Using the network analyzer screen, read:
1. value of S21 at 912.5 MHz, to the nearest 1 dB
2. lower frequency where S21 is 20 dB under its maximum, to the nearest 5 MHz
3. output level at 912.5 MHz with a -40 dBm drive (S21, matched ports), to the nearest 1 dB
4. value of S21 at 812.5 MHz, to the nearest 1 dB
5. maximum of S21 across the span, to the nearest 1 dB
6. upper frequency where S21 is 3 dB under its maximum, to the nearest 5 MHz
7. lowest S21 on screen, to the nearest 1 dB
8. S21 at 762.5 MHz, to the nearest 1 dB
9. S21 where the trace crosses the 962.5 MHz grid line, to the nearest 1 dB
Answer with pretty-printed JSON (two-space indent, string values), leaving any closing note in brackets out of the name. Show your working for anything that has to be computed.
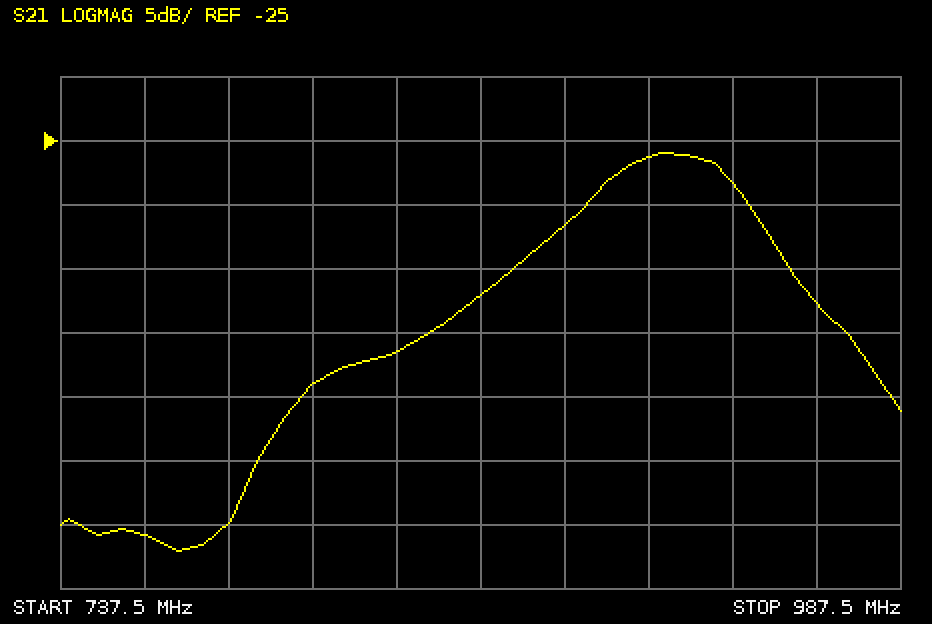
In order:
{
  "value of S21 at 912.5 MHz, to the nearest 1 dB": "-26 dB",
  "lower frequency where S21 is 20 dB under its maximum, to the nearest 5 MHz": "805 MHz",
  "output level at 912.5 MHz with a -40 dBm drive (S21, matched ports), to the nearest 1 dB": "-40 dBm + (-26 dB) = -66 dBm",
  "value of S21 at 812.5 MHz, to the nearest 1 dB": "-44 dB",
  "maximum of S21 across the span, to the nearest 1 dB": "-26 dB",
  "upper frequency where S21 is 3 dB under its maximum, to the nearest 5 MHz": "940 MHz",
  "lowest S21 on screen, to the nearest 1 dB": "-57 dB",
  "S21 at 762.5 MHz, to the nearest 1 dB": "-56 dB",
  "S21 where the trace crosses the 962.5 MHz grid line, to the nearest 1 dB": "-38 dB"
}
